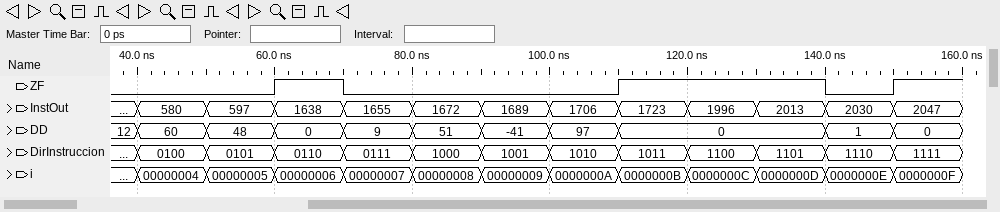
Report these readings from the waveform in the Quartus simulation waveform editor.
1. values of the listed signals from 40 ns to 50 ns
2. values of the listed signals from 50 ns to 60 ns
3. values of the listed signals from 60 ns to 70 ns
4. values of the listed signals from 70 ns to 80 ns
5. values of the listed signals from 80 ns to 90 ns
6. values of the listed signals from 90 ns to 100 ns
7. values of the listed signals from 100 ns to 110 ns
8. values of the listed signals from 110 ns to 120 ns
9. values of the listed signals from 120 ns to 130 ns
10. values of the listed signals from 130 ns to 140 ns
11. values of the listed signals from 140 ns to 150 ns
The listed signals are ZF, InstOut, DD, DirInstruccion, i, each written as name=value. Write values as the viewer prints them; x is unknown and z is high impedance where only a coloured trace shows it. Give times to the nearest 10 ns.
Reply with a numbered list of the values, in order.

1. ZF=0, InstOut=580, DD=60, DirInstruccion=0100, i=00000004
2. ZF=0, InstOut=597, DD=48, DirInstruccion=0101, i=00000005
3. ZF=1, InstOut=1638, DD=0, DirInstruccion=0110, i=00000006
4. ZF=0, InstOut=1655, DD=9, DirInstruccion=0111, i=00000007
5. ZF=0, InstOut=1672, DD=51, DirInstruccion=1000, i=00000008
6. ZF=0, InstOut=1689, DD=-41, DirInstruccion=1001, i=00000009
7. ZF=0, InstOut=1706, DD=97, DirInstruccion=1010, i=0000000A
8. ZF=1, InstOut=1723, DD=0, DirInstruccion=1011, i=0000000B
9. ZF=1, InstOut=1996, DD=0, DirInstruccion=1100, i=0000000C
10. ZF=1, InstOut=2013, DD=0, DirInstruccion=1101, i=0000000D
11. ZF=0, InstOut=2030, DD=1, DirInstruccion=1110, i=0000000E
